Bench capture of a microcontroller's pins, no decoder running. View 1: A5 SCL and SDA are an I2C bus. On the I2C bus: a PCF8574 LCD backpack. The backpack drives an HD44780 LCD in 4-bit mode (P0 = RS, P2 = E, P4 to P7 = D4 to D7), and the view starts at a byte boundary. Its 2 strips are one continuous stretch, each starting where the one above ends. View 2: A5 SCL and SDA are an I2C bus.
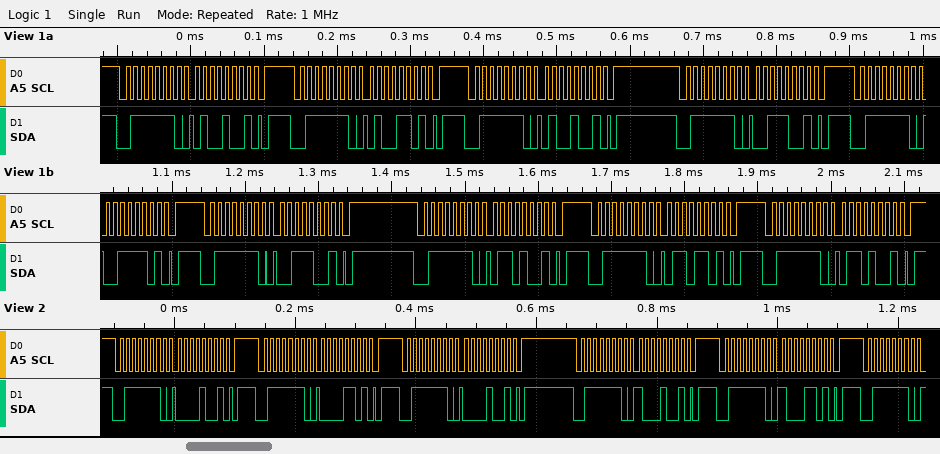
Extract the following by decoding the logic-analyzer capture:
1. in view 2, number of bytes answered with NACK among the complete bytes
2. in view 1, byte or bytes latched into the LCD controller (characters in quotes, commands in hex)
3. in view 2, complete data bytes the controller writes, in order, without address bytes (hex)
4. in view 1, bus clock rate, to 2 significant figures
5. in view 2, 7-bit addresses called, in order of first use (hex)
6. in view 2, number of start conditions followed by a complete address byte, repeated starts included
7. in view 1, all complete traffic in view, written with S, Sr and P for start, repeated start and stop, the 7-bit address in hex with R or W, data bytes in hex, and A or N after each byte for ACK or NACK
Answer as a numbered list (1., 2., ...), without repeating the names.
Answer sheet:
1. 0
2. 'C'
3. 09 0D 09 89 8D
4. 100 kHz
5. 0x3F
6. 6
7. S 3FW A 49 A P S 3FW A 4D A P S 3FW A 49 A P S 3FW A 39 A P S 3FW A 3D A P S 3FW A 39 A P S 3FW A 69 A P S 3FW A 6D A P S 3FW A 69 A P
